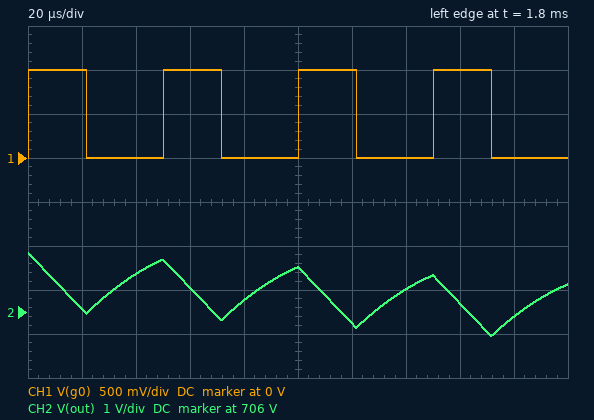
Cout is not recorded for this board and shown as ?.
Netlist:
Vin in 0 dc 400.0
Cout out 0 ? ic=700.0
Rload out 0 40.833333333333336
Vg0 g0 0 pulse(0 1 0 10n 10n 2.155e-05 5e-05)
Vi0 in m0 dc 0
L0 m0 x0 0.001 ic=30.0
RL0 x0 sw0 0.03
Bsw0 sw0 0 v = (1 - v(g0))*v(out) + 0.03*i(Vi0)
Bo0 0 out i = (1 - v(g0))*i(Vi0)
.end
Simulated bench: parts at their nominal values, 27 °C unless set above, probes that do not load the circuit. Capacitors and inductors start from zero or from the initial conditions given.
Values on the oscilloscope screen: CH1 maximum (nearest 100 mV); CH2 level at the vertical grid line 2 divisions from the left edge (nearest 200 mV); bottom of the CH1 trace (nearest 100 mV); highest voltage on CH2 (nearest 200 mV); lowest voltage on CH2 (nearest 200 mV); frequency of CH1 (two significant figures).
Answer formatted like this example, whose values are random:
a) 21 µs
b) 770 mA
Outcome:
a) 1.0 V
b) 706.8 V
c) 0 V
d) 707.4 V
e) 705.4 V
f) 20 kHz
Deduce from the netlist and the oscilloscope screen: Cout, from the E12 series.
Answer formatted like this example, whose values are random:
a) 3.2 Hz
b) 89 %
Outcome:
a) 270 µF
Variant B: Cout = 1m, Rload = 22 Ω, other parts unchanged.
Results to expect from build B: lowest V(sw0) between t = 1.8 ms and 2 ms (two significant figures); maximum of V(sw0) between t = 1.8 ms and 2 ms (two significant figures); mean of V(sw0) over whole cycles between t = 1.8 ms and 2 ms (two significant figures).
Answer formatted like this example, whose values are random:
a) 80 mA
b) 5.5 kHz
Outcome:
a) 1.2 V
b) 680 V
c) 390 V
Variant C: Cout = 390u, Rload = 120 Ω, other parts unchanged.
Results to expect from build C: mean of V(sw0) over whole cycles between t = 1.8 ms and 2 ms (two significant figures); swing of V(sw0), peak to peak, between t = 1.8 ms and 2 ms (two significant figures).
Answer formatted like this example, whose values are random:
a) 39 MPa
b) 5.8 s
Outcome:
a) 420 V
b) 740 V
